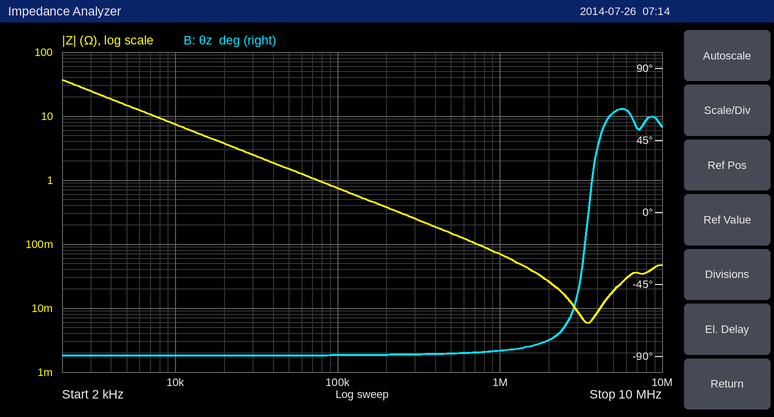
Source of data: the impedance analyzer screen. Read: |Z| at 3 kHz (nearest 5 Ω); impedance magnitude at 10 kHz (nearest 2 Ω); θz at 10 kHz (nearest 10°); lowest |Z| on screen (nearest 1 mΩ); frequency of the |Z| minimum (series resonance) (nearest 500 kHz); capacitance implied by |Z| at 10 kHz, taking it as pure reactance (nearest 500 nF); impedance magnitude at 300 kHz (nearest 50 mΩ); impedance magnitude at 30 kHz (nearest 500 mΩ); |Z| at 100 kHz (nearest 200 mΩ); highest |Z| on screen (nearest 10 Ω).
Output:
25 Ω
8 Ω
-90°
6 mΩ
3.5 MHz
2.0 µF
250 mΩ
2.5 Ω
800 mΩ
40 Ω
